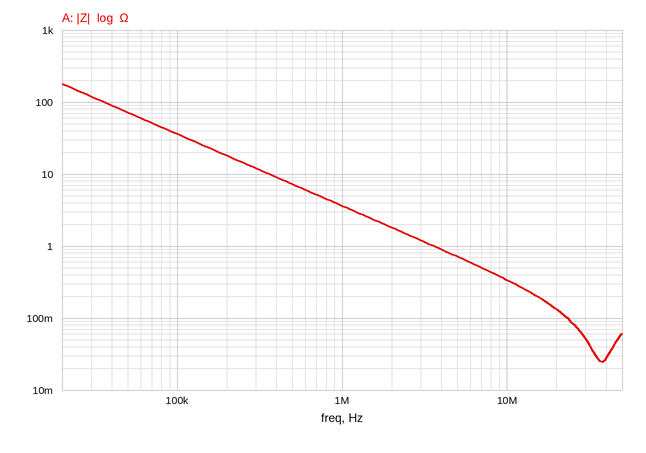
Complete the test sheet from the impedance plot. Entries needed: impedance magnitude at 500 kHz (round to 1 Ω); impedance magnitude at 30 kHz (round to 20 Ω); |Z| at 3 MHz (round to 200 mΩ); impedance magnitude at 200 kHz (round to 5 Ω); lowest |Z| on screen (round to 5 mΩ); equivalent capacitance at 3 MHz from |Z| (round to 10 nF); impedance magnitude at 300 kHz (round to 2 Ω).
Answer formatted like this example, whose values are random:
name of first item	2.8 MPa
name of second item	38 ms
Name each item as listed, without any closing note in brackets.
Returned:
impedance magnitude at 500 kHz	7 Ω
impedance magnitude at 30 kHz	120 Ω
|Z| at 3 MHz	1.2 Ω
impedance magnitude at 200 kHz	20 Ω
lowest |Z| on screen	25 mΩ
equivalent capacitance at 3 MHz from |Z|	40 nF
impedance magnitude at 300 kHz	12 Ω
